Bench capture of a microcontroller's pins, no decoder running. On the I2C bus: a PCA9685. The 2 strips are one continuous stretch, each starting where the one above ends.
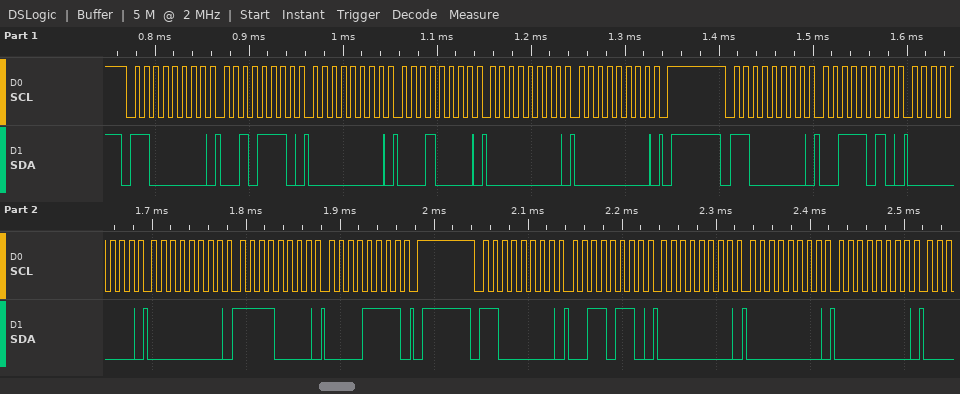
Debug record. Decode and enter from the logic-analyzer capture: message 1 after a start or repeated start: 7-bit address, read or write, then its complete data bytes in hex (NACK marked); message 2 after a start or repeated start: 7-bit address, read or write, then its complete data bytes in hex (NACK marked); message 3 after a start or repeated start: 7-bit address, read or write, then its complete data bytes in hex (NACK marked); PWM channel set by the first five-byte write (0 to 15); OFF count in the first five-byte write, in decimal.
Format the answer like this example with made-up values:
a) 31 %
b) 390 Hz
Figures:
a) 0x60 write: 2E 00 10 00 00
b) 0x60 write: 3A 00 00 F0 0F
c) 0x60 write: 36 00 00 00
d) 10
e) 0
